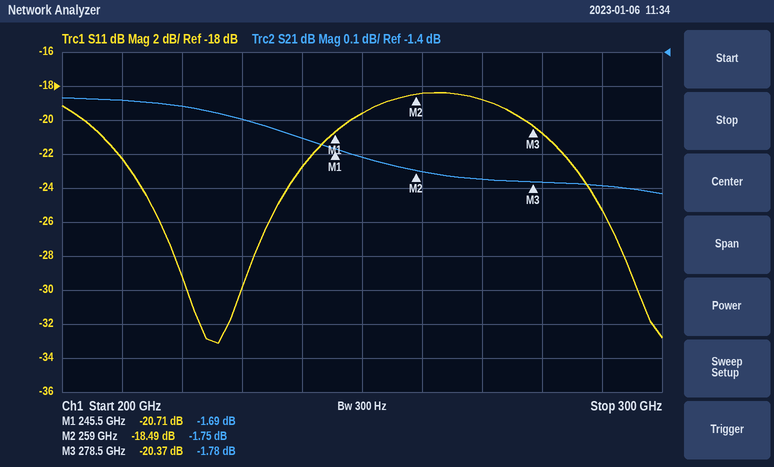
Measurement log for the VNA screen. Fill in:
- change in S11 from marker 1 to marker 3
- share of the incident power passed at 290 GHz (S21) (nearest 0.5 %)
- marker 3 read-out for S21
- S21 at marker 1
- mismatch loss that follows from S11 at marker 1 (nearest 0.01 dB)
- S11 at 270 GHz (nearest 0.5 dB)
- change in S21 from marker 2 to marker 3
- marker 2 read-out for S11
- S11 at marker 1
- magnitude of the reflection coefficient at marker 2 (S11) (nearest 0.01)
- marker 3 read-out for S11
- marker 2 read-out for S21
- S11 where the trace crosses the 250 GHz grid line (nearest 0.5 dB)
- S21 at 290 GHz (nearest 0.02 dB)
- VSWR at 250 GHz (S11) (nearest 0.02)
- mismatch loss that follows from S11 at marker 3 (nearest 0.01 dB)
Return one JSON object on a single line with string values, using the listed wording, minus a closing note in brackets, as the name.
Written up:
{"change in S11 from marker 1 to marker 3": "0.34 dB", "share of the incident power passed at 290 GHz (S21)": "66.0 %", "marker 3 read-out for S21": "-1.78 dB", "S21 at marker 1": "-1.69 dB", "mismatch loss that follows from S11 at marker 1": "0.04 dB", "S11 at 270 GHz": "-19.0 dB", "change in S21 from marker 2 to marker 3": "-0.03 dB", "marker 2 read-out for S11": "-18.49 dB", "S11 at marker 1": "-20.71 dB", "magnitude of the reflection coefficient at marker 2 (S11)": "0.12", "marker 3 read-out for S11": "-20.37 dB", "marker 2 read-out for S21": "-1.75 dB", "S11 where the trace crosses the 250 GHz grid line": "-19.5 dB", "S21 at 290 GHz": "-1.80 dB", "VSWR at 250 GHz (S11)": "1.24", "mismatch loss that follows from S11 at marker 3": "0.04 dB"}
